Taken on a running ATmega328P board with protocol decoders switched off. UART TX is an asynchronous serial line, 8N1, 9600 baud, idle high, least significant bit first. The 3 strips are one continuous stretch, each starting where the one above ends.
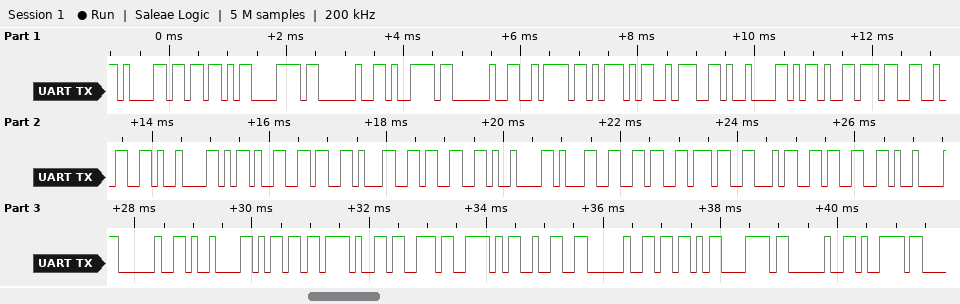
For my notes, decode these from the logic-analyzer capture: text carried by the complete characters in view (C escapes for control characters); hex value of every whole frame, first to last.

"a[x y z]:\t-72\t-613\t16743\t \tm/s^2 [x y"
0x61 0x5B 0x78 0x20 0x79 0x20 0x7A 0x5D 0x3A 0x09 0x2D 0x37 0x32 0x09 0x2D 0x36 0x31 0x33 0x09 0x31 0x36 0x37 0x34 0x33 0x09 0x20 0x09 0x6D 0x2F 0x73 0x5E 0x32 0x20 0x5B 0x78 0x20 0x79
